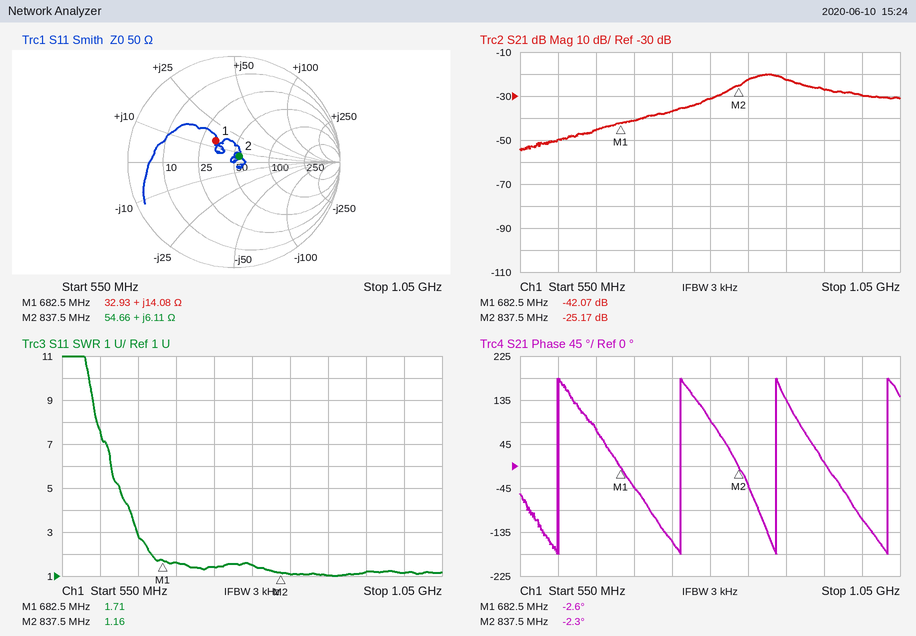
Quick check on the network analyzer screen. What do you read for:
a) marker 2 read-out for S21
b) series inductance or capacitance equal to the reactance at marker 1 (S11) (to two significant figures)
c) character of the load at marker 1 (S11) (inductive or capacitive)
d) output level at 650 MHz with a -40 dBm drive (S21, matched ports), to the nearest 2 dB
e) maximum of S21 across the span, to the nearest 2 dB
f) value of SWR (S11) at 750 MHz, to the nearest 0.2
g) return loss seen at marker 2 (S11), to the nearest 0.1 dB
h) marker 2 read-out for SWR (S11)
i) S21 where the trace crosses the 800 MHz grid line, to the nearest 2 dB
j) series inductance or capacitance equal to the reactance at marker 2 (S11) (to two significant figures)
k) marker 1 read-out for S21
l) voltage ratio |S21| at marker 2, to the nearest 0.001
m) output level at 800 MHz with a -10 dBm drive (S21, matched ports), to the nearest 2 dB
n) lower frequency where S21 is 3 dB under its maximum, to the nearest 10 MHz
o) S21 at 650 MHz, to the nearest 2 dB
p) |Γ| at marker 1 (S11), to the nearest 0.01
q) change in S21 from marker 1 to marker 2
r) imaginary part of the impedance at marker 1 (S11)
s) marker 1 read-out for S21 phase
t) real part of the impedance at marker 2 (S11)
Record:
-25.17 dB
3.3 nH
inductive
-86 dBm
-20 dB
1.4
22.7 dB
1.16
-32 dB
1.2 nH
-42.07 dB
0.055
-42 dBm
850 MHz
-46 dB
0.26
16.90 dB
+14.08 Ω
-2.6°
54.66 Ω
